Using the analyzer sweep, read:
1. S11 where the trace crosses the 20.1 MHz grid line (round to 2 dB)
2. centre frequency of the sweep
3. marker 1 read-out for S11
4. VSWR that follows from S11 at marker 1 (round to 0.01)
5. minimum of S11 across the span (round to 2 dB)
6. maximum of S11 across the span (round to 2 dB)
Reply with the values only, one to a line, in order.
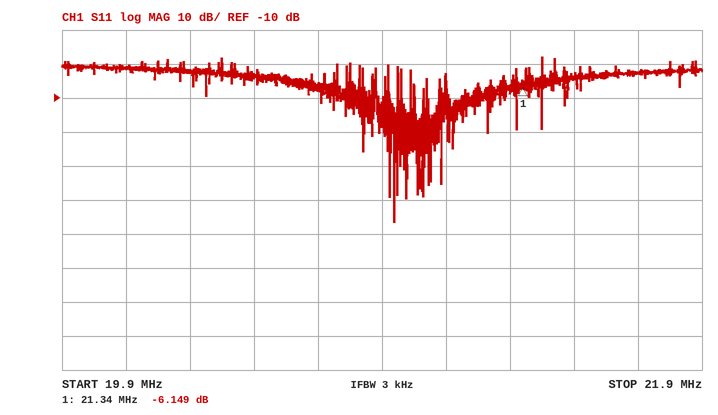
-2 dB
20.9 MHz
-6.149 dB
2.94
-46 dB
2 dB
